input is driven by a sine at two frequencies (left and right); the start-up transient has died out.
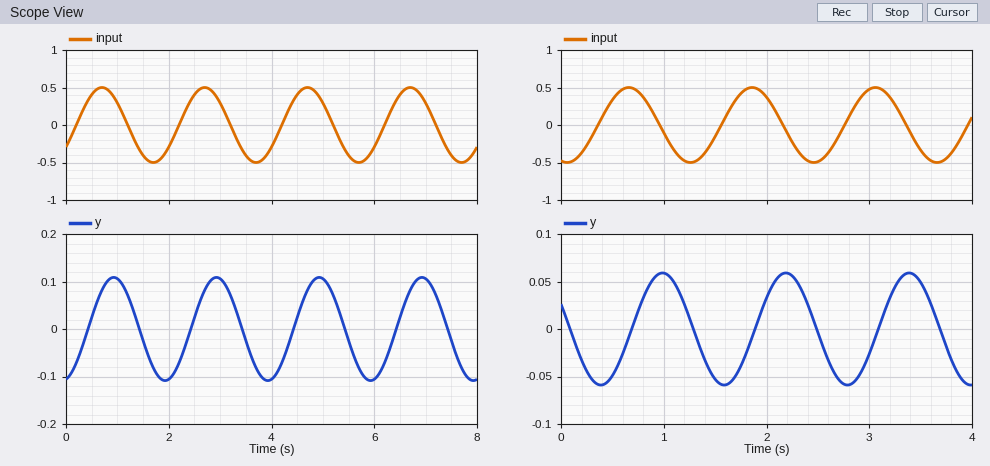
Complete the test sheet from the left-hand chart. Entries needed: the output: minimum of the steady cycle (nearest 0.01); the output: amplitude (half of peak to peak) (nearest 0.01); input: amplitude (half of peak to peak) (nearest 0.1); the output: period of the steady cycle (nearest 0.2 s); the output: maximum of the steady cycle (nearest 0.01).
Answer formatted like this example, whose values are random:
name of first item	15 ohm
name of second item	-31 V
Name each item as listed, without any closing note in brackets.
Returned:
the output: minimum of the steady cycle	-0.11
the output: amplitude (half of peak to peak)	0.11
input: amplitude (half of peak to peak)	0.5
the output: period of the steady cycle	2.0 s
the output: maximum of the steady cycle	0.11
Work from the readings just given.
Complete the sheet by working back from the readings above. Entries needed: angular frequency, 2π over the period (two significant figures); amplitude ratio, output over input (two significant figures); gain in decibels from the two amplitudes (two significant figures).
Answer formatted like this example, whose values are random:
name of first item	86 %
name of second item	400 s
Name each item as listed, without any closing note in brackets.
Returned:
angular frequency, 2π over the period	3.1 rad/s
amplitude ratio, output over input	0.22
gain in decibels from the two amplitudes	-13 dB
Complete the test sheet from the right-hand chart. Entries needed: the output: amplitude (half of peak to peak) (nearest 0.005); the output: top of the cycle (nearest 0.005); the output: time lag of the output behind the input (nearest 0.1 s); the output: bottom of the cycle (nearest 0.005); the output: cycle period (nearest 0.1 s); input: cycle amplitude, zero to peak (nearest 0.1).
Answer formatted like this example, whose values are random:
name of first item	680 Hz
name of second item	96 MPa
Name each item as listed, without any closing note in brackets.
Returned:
the output: amplitude (half of peak to peak)	0.060
the output: top of the cycle	0.060
the output: time lag of the output behind the input	0.3 s
the output: bottom of the cycle	-0.060
the output: cycle period	1.2 s
input: cycle amplitude, zero to peak	0.5
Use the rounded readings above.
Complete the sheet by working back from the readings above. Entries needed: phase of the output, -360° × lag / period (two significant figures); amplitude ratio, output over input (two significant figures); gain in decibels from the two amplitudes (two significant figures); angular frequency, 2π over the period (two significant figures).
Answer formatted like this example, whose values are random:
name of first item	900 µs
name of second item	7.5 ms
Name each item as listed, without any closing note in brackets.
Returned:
phase of the output, -360° × lag / period	-90°
amplitude ratio, output over input	0.12
gain in decibels from the two amplitudes	-18 dB
angular frequency, 2π over the period	5.2 rad/s
